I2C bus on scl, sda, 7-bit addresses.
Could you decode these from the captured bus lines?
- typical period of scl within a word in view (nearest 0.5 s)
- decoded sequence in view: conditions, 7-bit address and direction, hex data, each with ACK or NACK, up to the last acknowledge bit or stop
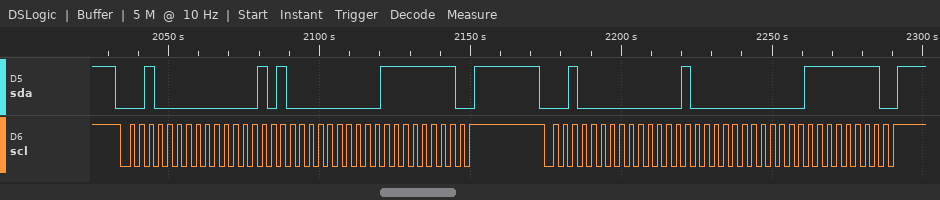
3 s
start, address 10 write ACK, 05 ACK, 00 ACK, FF ACK, stop, start, address 10 write ACK, 04 ACK, 00 ACK, FF ACK, stop
